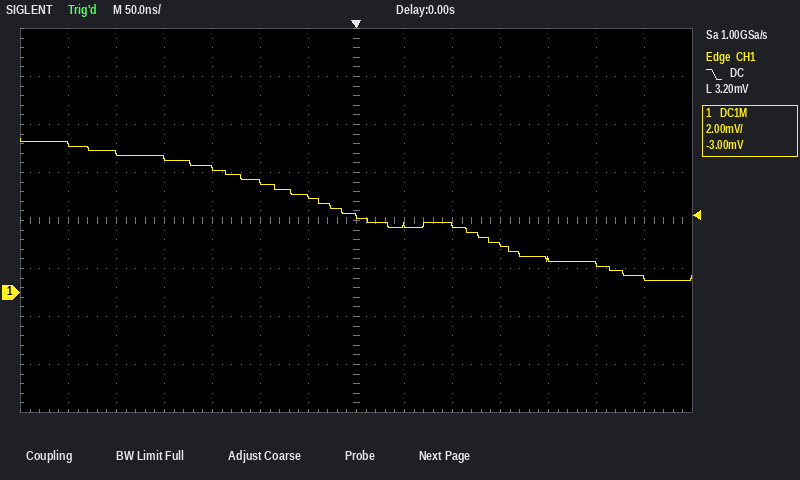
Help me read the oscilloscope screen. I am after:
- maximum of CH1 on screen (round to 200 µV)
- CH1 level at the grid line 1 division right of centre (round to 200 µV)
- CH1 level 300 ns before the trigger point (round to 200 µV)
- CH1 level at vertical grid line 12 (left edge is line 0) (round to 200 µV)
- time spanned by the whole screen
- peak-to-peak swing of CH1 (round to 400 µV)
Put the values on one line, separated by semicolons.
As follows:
6.4 mV; 2.8 mV; 6.2 mV; 1.2 mV; 700 ns; 6.0 mV
